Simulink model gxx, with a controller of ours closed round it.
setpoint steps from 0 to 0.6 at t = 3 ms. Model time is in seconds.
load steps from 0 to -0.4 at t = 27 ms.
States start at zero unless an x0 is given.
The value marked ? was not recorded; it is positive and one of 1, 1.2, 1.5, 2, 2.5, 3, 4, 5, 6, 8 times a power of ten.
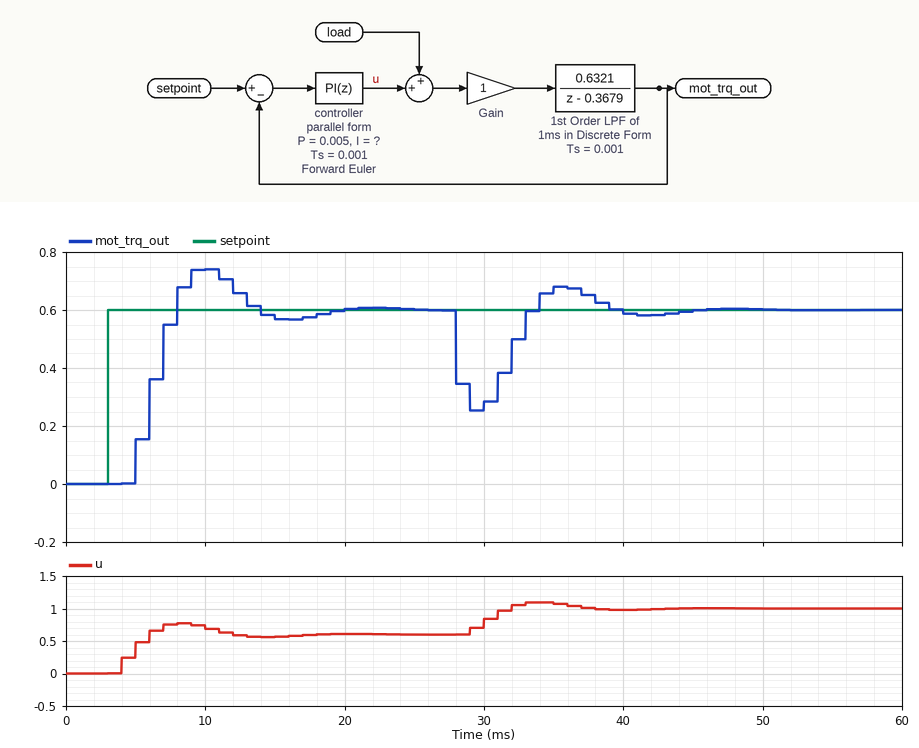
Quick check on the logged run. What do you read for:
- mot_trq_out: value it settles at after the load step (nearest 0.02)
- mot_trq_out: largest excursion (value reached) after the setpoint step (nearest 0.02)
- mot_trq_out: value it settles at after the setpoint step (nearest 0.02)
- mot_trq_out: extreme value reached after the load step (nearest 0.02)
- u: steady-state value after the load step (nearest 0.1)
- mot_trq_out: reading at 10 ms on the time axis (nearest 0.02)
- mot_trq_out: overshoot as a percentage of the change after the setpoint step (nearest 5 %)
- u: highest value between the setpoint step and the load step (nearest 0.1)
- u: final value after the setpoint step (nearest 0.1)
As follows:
0.60
0.74
0.60
0.26
1.0
0.74
25 %
0.8
0.6
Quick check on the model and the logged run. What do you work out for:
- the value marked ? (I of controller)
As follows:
400
